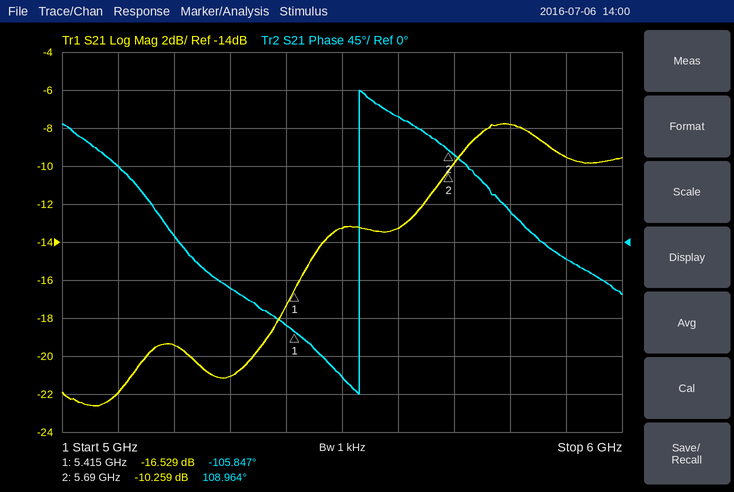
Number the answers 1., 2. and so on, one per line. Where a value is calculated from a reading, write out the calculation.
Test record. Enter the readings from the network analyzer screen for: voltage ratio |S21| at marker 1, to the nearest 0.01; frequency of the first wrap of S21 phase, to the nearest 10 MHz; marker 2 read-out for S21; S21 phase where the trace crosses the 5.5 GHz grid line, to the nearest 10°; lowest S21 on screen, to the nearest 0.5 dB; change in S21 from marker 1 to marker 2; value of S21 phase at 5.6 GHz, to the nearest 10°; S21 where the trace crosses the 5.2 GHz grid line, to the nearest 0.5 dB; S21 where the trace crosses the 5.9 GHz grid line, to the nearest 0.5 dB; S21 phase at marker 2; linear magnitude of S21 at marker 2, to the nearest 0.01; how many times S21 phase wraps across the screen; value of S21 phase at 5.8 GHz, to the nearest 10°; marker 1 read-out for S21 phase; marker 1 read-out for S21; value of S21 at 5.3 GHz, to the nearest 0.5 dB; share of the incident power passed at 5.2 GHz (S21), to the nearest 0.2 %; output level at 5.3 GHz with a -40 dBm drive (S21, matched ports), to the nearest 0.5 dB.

1. 10^(-16.529/20) ≈ 0.15
2. 5.53 GHz
3. -10.259 dB
4. -160°
5. -22.5 dB
6. -10.259 − (-16.529) = 6.270 dB
7. 150°
8. -19.5 dB
9. -9.5 dB
10. 108.964°
11. 10^(-10.259/20) ≈ 0.31
12. 1
13. 40°
14. -105.847°
15. -16.529 dB
16. -21.0 dB
17. 10^(-19.5/10) ≈ 1.12 %, so 1.2 % to the nearest 0.2 %
18. -40 dBm + (-21.0 dB) = -61.0 dBm
